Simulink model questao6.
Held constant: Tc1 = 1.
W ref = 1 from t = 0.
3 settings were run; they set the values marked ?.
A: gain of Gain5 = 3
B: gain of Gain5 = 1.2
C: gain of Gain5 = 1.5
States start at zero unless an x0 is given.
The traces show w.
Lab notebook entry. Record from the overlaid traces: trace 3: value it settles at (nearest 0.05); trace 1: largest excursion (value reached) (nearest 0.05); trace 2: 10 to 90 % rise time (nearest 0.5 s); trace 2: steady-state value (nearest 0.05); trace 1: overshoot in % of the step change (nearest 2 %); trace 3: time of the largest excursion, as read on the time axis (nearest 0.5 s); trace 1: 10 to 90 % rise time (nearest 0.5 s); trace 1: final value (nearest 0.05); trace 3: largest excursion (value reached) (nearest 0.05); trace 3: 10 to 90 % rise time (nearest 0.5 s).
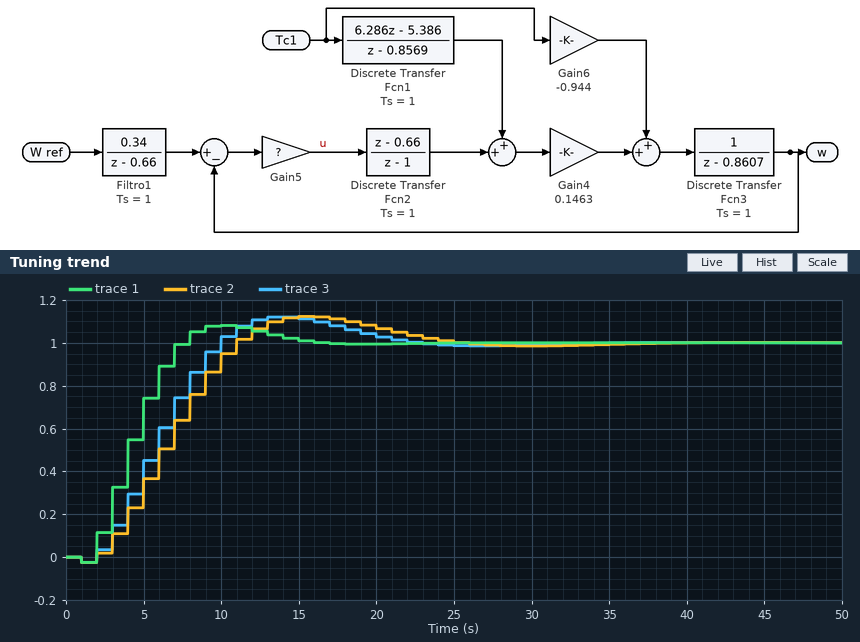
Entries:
1.00
1.10
7.0 s
1.00
8 %
14.0 s
5.0 s
1.00
1.10
6.0 s
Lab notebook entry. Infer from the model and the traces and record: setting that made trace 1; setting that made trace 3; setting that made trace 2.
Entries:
A
C
B
